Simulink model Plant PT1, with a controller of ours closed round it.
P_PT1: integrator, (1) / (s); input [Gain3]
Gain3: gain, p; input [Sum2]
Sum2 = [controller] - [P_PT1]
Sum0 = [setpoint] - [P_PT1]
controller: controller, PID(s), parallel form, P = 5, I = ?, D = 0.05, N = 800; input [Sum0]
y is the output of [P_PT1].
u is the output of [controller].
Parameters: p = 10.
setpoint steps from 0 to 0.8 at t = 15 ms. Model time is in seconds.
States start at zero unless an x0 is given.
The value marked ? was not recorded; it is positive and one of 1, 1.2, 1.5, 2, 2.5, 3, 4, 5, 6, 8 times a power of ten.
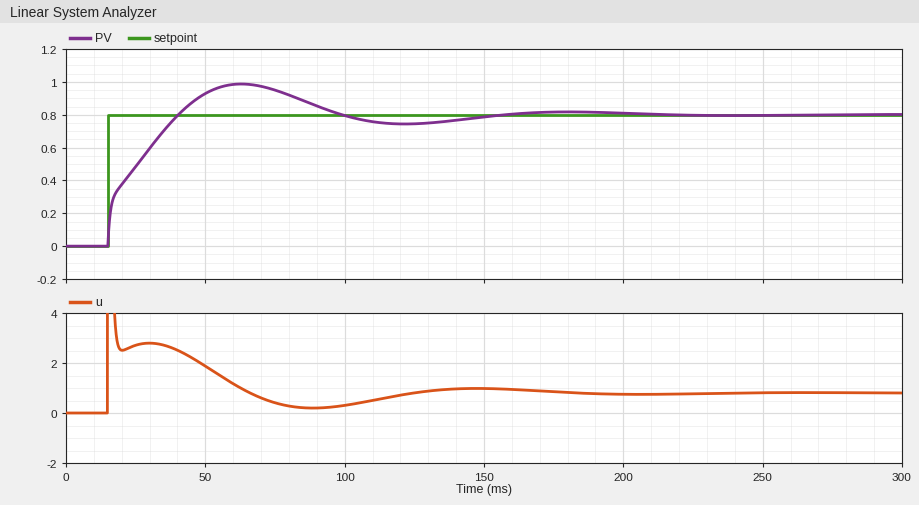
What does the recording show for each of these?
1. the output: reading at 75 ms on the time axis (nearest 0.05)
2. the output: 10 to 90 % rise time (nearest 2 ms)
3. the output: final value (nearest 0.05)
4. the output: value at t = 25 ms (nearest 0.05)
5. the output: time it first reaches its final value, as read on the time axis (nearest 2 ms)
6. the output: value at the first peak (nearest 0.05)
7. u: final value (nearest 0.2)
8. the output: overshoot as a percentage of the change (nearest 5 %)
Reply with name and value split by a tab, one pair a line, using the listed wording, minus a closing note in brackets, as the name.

the output: reading at 75 ms on the time axis	0.95
the output: 10 to 90 % rise time	20 ms
the output: final value	0.80
the output: value at t = 25 ms	0.50
the output: time it first reaches its final value, as read on the time axis	40 ms
the output: value at the first peak	1.00
u: final value	0.8
the output: overshoot as a percentage of the change	25 %
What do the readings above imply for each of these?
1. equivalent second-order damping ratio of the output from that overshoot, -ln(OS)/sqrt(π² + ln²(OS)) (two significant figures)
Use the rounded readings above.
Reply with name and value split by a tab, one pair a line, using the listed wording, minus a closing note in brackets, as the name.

equivalent second-order damping ratio of the output from that overshoot, -ln(OS)/sqrt(π² + ln²(OS))	0.40
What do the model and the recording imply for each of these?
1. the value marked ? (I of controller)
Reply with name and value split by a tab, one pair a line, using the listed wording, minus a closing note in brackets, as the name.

the value marked ?	500
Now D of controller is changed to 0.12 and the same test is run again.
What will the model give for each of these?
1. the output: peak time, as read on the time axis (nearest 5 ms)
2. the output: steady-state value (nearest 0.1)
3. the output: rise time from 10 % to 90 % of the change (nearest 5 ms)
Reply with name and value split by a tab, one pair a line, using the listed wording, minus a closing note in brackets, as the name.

the output: peak time, as read on the time axis	75 ms
the output: steady-state value	0.8
the output: rise time from 10 % to 90 % of the change	25 ms
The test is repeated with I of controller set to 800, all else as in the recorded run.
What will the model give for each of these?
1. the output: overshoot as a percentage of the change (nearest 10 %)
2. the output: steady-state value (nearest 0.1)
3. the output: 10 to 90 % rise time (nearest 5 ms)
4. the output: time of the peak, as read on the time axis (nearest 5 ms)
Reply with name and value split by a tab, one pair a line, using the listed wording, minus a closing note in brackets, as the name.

the output: overshoot as a percentage of the change	30 %
the output: steady-state value	0.8
the output: 10 to 90 % rise time	15 ms
the output: time of the peak, as read on the time axis	55 ms
